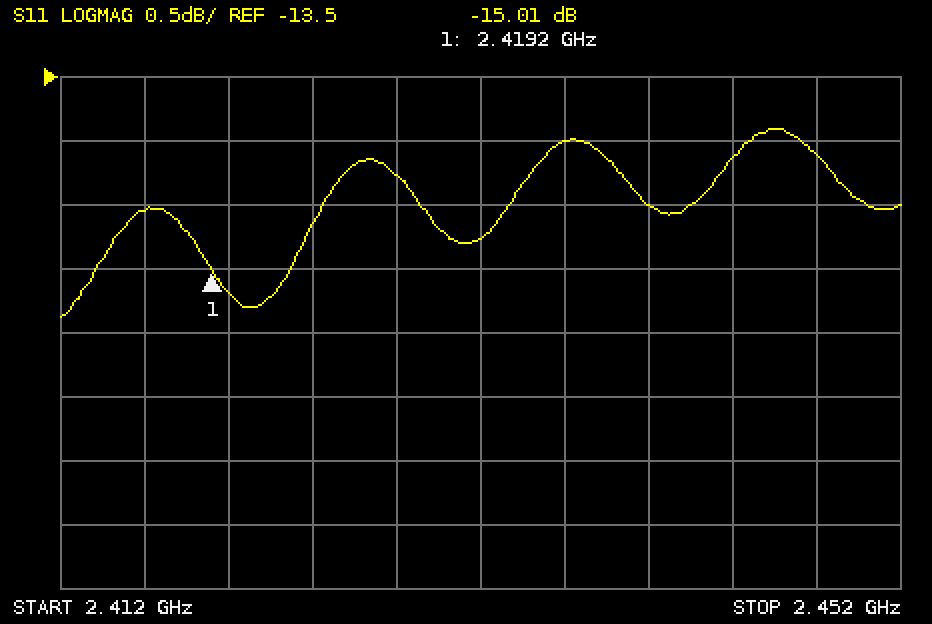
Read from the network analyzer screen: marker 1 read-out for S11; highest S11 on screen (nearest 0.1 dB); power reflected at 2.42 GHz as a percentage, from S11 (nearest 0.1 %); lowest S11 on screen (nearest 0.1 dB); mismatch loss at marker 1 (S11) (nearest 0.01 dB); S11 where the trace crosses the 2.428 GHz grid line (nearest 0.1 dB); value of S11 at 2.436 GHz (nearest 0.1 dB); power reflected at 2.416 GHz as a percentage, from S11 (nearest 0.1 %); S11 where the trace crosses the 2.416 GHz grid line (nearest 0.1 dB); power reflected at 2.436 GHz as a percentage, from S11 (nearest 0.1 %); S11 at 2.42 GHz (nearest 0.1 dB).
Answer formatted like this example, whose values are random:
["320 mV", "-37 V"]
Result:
["-15.01 dB", "-13.9 dB", "3.0 %", "-15.4 dB", "0.14 dB", "-14.3 dB", "-14.0 dB", "3.5 %", "-14.5 dB", "4.0 %", "-15.2 dB"]
